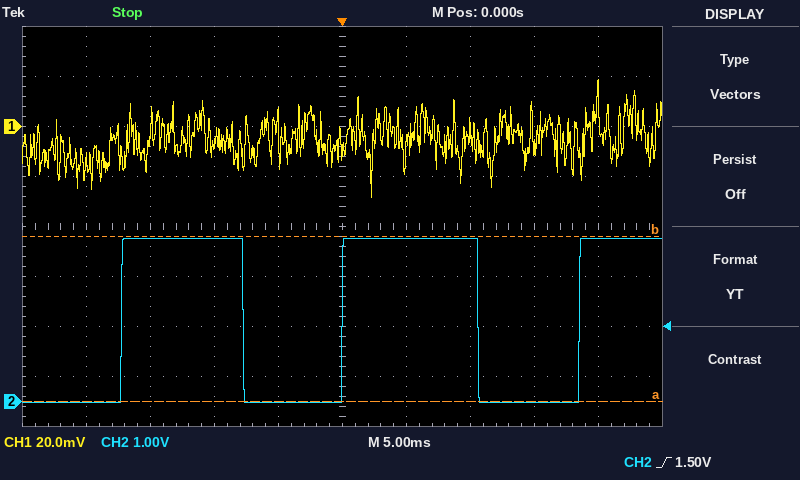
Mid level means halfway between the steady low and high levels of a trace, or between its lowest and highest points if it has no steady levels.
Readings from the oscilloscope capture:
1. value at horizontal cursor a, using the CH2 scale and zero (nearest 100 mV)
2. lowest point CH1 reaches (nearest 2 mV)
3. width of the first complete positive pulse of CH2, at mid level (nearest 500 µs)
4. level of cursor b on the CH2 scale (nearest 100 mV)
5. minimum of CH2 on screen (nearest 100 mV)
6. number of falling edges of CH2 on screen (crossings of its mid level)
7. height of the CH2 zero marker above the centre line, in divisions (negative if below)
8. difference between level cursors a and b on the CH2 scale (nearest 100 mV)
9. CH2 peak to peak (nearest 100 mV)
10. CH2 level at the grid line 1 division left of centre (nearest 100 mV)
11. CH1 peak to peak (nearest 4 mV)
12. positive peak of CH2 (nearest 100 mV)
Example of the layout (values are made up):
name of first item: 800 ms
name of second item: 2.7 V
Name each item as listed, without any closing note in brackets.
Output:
value at horizontal cursor a, using the CH2 scale and zero: 0.0 V
lowest point CH1 reaches: -28 mV
width of the first complete positive pulse of CH2, at mid level: 9.5 ms
level of cursor b on the CH2 scale: 3.3 V
minimum of CH2 on screen: 0.0 V
number of falling edges of CH2 on screen: 2
height of the CH2 zero marker above the centre line, in divisions: -3.5 div
difference between level cursors a and b on the CH2 scale: 3.3 V
CH2 peak to peak: 3.3 V
CH2 level at the grid line 1 division left of centre: 0.0 V
CH1 peak to peak: 48 mV
positive peak of CH2: 3.3 V
